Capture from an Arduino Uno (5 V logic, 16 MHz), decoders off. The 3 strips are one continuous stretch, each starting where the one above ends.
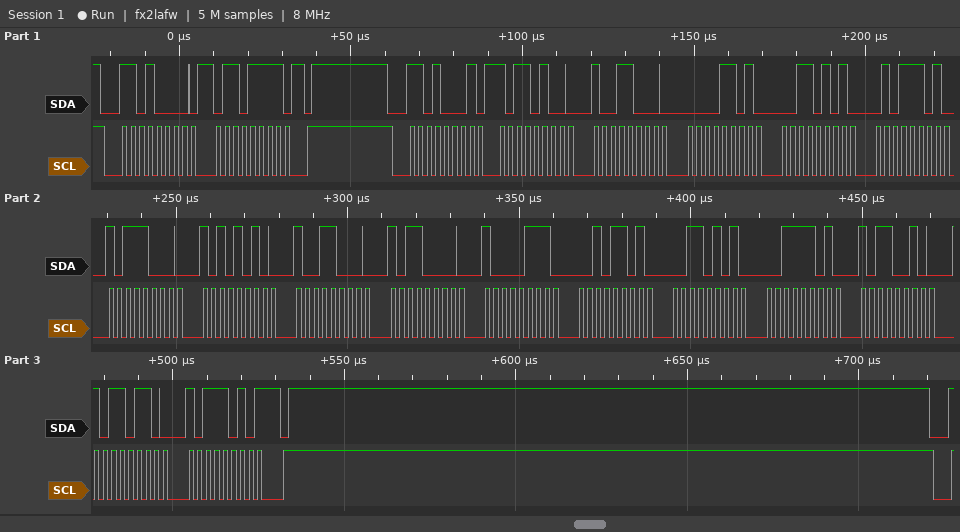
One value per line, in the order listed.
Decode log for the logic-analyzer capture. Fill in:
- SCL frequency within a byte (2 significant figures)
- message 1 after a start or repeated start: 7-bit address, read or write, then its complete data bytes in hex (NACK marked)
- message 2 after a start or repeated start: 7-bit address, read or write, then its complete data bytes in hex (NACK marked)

400 kHz
0x68 write: 6F
0x68 read: B4 98 0D 35 5D B8 AA 98 B0 87 2D 35 3D B2 B6 BA NACK
